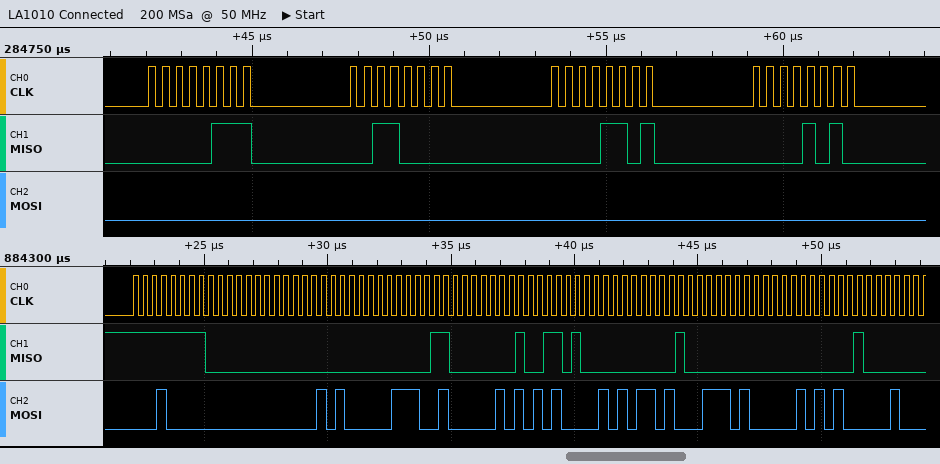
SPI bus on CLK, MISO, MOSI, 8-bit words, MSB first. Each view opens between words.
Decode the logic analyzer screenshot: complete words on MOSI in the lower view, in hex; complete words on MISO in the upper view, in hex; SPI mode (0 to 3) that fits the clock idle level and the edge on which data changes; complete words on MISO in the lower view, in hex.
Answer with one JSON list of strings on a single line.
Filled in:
["10, 00, 0A, 0E, 41, 54, 2B, 47, 41, 50", "07, 30, 0D, 0A", "0", "FF, 00, 00, 00, C0, 4D, 00, 20, 00, 04"]
